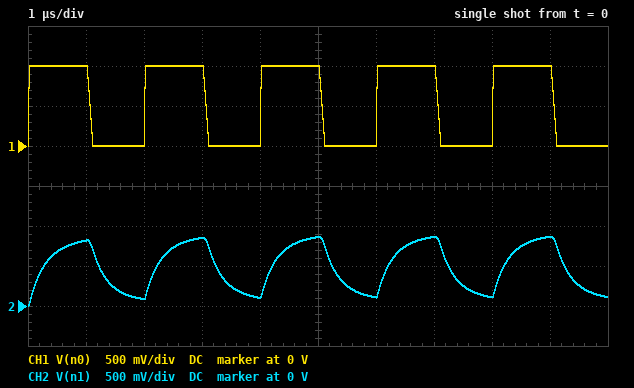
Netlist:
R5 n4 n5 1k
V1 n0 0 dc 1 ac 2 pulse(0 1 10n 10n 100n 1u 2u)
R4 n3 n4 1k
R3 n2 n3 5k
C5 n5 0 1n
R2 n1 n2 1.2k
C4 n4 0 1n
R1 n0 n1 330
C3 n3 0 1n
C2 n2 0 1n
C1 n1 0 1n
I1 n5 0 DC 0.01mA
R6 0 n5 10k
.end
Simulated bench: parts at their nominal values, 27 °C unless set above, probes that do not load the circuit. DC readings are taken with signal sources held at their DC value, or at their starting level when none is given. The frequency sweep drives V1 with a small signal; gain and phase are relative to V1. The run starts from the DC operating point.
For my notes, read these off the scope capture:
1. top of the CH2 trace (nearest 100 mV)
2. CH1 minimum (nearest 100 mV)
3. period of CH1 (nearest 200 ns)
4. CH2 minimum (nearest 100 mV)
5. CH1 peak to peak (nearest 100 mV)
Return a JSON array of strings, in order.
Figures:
["900 mV", "0 V", "2.0 µs", "0 V", "1.0 V"]
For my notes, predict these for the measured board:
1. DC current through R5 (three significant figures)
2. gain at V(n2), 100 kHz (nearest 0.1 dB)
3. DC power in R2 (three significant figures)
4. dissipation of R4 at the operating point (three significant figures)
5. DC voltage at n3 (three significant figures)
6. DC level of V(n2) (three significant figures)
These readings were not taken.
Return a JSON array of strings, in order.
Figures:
["59.4 µA", "-4.5 dB", "4.23 µW", "3.52 µW", "612 mV", "909 mV"]
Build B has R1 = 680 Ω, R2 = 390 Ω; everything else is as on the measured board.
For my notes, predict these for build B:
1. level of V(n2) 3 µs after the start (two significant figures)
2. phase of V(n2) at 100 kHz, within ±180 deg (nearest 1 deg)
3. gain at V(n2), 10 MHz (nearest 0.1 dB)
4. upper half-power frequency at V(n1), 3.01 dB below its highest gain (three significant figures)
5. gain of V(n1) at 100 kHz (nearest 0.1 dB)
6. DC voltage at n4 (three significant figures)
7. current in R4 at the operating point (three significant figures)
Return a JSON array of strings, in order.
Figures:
["500 mV", "-47 deg", "-60.4 dB", "105 kHz", "-3.2 dB", "570 mV", "60.9 µA"]
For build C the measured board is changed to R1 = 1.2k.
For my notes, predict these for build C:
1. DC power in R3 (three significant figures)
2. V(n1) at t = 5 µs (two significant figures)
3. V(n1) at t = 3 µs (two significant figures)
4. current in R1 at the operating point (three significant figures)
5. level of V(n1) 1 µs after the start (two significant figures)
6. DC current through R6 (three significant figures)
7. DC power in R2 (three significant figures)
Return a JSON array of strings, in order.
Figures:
["16.1 µW", "570 mV", "530 mV", "56.7 µA", "430 mV", "46.7 µA", "3.86 µW"]
